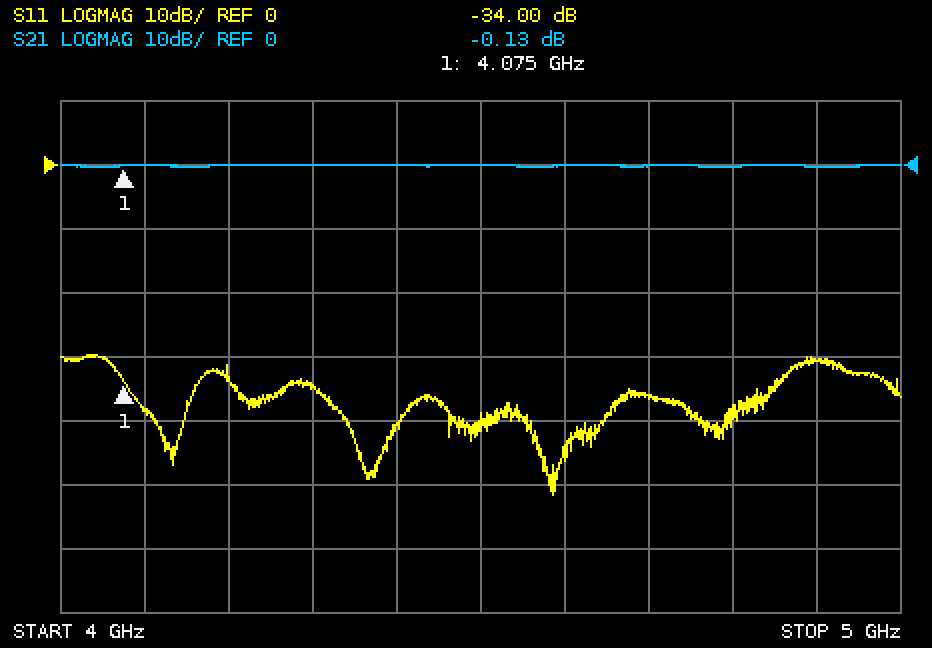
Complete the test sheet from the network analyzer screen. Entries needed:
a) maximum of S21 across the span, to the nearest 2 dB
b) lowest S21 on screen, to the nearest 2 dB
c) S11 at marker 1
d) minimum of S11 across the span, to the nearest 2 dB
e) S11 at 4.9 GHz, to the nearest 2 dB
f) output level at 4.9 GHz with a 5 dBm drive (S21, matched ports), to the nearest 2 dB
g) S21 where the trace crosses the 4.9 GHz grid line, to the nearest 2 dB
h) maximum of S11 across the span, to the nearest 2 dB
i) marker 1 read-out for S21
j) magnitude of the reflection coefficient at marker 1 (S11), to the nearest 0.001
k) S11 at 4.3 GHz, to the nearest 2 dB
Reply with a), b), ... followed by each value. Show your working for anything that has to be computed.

a) 0 dB
b) 0 dB
c) -34.00 dB
d) -52 dB
e) -30 dB
f) 5 dBm + (0 dB) = 4 dBm
g) 0 dB
h) -30 dB
i) -0.13 dB
j) 10^(-34/20) ≈ 0.020
k) -34 dB
